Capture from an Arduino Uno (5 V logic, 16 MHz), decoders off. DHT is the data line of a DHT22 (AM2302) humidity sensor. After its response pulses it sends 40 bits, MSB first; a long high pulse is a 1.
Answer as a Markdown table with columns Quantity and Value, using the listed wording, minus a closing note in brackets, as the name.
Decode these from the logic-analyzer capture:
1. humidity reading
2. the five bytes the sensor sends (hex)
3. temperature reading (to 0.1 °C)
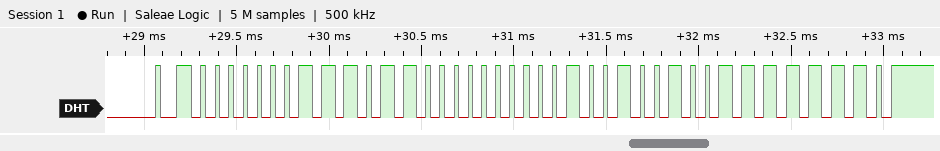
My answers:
| Quantity | Value |
|---|---|
| humidity reading | 47.2 % |
| the five bytes the sensor sends | 01 D8 01 24 FE |
| temperature reading | 29.2 °C |
